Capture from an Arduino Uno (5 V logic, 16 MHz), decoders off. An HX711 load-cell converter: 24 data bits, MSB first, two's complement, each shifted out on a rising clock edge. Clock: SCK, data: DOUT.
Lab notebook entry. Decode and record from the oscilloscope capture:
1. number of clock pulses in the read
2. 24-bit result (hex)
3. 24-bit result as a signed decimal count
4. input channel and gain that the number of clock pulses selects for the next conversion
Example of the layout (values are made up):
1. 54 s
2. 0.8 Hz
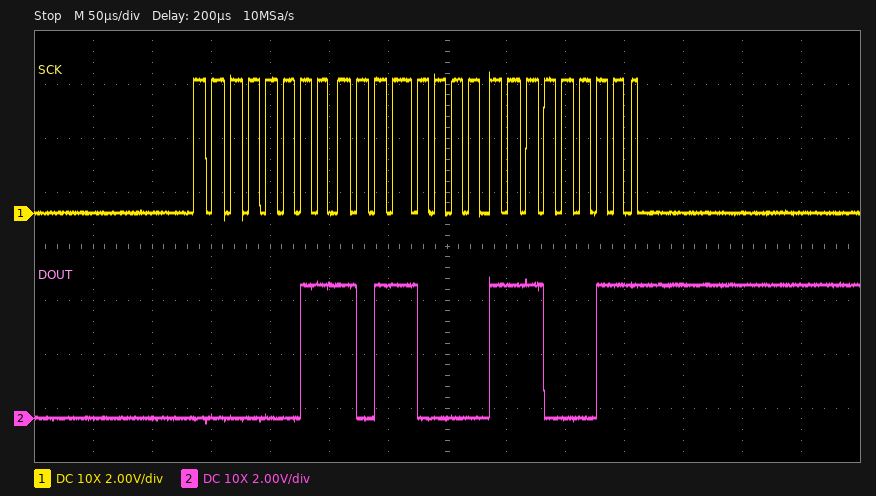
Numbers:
1. 25
2. 0x03B0E3
3. 241891
4. channel A, gain 128
